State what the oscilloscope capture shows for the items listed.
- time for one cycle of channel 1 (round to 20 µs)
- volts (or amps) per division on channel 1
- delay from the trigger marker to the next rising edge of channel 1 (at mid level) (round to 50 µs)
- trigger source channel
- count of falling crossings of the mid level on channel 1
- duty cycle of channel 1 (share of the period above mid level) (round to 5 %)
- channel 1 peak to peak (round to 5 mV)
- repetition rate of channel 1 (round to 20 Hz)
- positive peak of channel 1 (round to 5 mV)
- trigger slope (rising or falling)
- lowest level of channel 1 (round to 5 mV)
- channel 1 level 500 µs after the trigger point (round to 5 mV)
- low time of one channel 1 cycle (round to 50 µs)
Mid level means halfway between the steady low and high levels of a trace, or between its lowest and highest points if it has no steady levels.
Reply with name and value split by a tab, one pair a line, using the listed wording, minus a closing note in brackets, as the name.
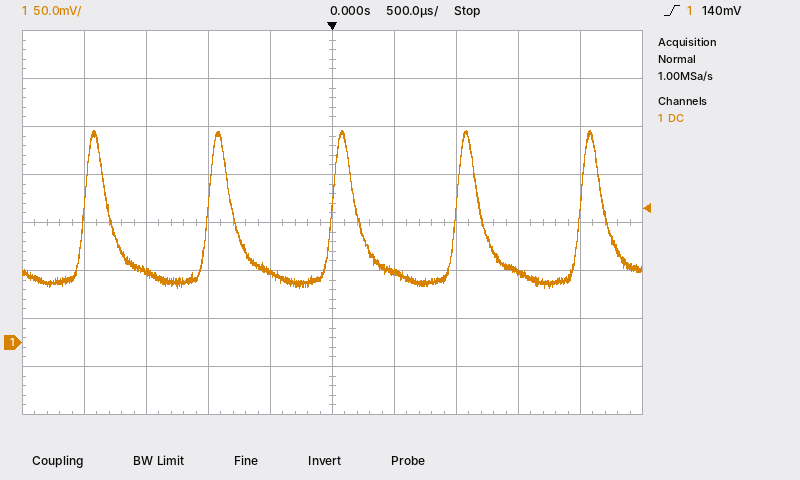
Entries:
time for one cycle of channel 1	1.00 ms
volts (or amps) per division on channel 1	50 mV
delay from the trigger marker to the next rising edge of channel 1 (at mid level)	1.00 ms
trigger source channel	channel 1
count of falling crossings of the mid level on channel 1	5
duty cycle of channel 1 (share of the period above mid level)	20 %
channel 1 peak to peak	165 mV
repetition rate of channel 1	1.00 kHz
positive peak of channel 1	220 mV
trigger slope	rising
lowest level of channel 1	55 mV
channel 1 level 500 µs after the trigger point	75 mV
low time of one channel 1 cycle	800 µs
